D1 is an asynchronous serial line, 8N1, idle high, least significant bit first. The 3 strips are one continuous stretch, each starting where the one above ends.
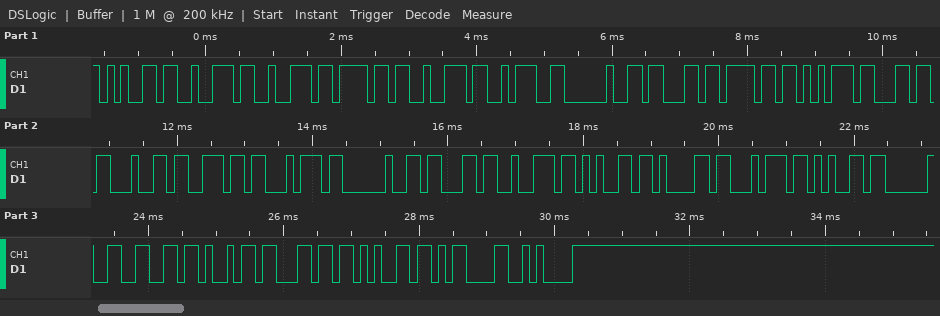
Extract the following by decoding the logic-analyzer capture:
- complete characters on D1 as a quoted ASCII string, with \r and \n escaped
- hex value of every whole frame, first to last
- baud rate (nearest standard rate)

"error: couldnt create file\r\n"
65 72 72 6F 72 3A 20 63 6F 75 6C 64 6E 74 20 63 72 65 61 74 65 20 66 69 6C 65 0D 0A
9600 baud
